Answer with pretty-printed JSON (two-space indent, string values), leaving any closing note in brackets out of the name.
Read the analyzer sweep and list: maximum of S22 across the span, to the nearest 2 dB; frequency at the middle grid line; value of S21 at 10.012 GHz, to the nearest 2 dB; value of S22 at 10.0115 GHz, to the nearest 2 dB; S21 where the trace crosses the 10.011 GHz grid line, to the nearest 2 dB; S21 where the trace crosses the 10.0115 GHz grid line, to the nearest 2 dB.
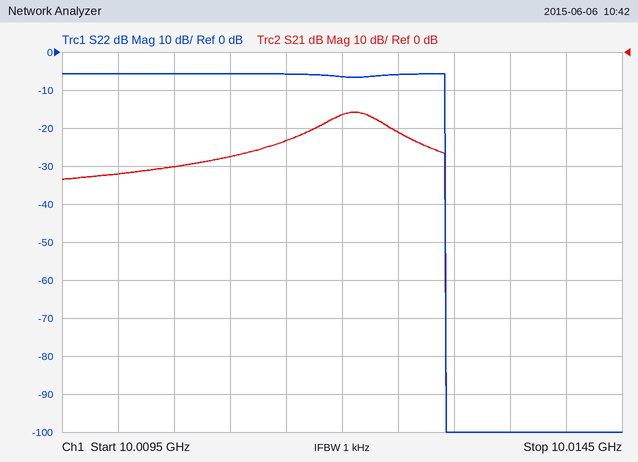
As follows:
{
  "maximum of S22 across the span, to the nearest 2 dB": "-6 dB",
  "frequency at the middle grid line": "10.012 GHz",
  "value of S21 at 10.012 GHz, to the nearest 2 dB": "-16 dB",
  "value of S22 at 10.0115 GHz, to the nearest 2 dB": "-6 dB",
  "S21 where the trace crosses the 10.011 GHz grid line, to the nearest 2 dB": "-28 dB",
  "S21 where the trace crosses the 10.0115 GHz grid line, to the nearest 2 dB": "-24 dB"
}
